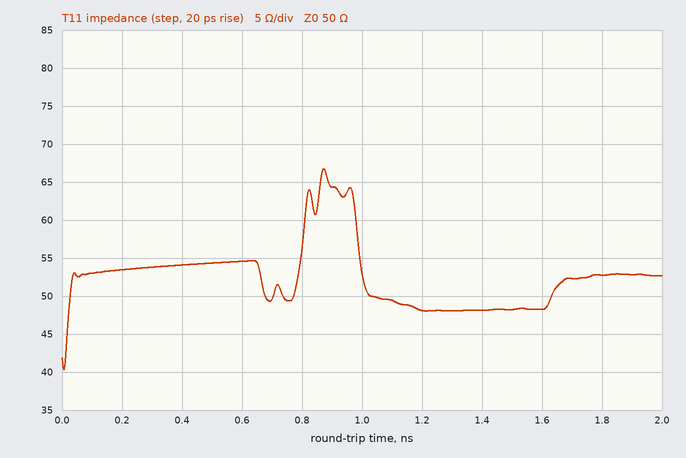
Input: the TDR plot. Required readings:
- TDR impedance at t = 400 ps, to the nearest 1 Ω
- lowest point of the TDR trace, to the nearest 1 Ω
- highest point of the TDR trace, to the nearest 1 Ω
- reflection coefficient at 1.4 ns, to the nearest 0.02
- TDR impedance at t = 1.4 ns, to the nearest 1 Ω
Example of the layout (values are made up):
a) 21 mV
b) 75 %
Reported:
a) 54 Ω
b) 40 Ω
c) 67 Ω
d) -0.02
e) 48 Ω
